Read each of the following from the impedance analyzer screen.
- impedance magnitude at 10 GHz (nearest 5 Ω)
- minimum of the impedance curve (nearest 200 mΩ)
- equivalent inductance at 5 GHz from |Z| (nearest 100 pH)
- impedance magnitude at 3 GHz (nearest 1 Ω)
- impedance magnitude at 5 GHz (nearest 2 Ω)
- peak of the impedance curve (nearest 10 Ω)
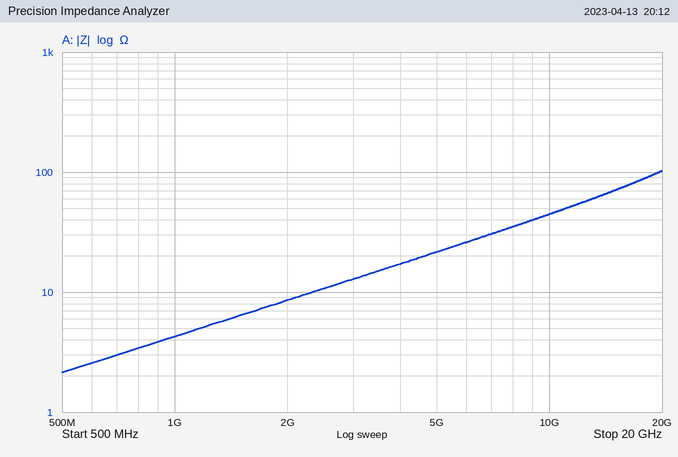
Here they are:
45 Ω
2.2 Ω
700 pH
13 Ω
22 Ω
100 Ω
